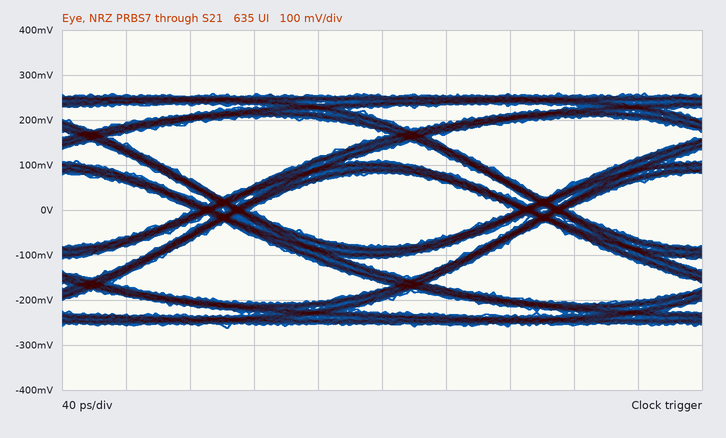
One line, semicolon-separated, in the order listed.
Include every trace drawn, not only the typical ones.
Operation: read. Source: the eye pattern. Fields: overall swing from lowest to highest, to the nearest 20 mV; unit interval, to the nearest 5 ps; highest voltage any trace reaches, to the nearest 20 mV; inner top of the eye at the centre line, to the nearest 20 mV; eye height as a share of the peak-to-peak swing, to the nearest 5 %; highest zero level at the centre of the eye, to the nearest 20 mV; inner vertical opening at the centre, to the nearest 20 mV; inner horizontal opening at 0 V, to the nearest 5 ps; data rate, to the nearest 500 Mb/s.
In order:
520 mV; 200 ps; 260 mV; 80 mV; 30 %; -80 mV; 160 mV; 165 ps; 5.0 Gb/s
